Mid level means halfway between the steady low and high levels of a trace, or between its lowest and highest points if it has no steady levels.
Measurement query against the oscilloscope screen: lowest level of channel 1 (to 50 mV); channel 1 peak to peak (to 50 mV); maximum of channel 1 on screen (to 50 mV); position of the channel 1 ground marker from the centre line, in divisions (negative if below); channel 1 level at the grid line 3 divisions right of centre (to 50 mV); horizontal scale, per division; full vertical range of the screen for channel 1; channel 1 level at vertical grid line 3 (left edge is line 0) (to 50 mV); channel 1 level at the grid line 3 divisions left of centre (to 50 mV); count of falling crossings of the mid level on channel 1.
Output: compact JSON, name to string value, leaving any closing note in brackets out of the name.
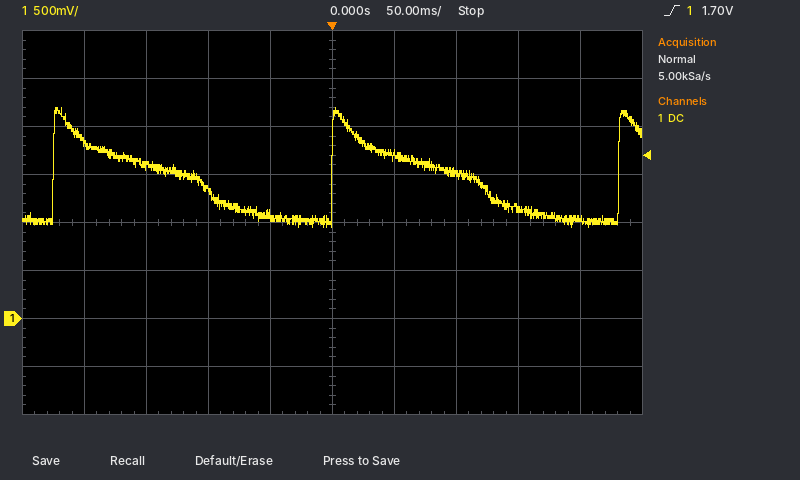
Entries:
{"lowest level of channel 1": "950 mV", "channel 1 peak to peak": "1.25 V", "maximum of channel 1 on screen": "2.20 V", "position of the channel 1 ground marker from the centre line, in divisions": "-2.0 div", "channel 1 level at the grid line 3 divisions right of centre": "1.15 V", "horizontal scale, per division": "50 ms", "full vertical range of the screen for channel 1": "4 V", "channel 1 level at vertical grid line 3 (left edge is line 0)": "1.35 V", "channel 1 level at the grid line 3 divisions left of centre": "1.60 V", "count of falling crossings of the mid level on channel 1": "2"}
